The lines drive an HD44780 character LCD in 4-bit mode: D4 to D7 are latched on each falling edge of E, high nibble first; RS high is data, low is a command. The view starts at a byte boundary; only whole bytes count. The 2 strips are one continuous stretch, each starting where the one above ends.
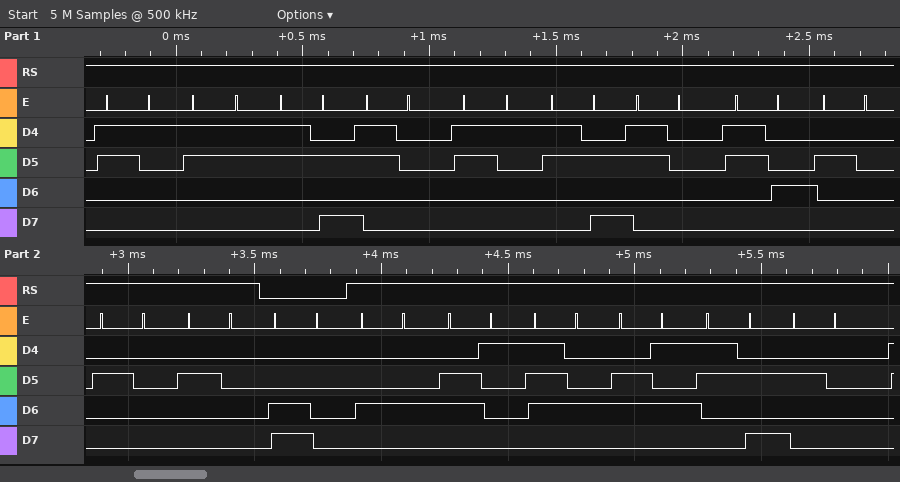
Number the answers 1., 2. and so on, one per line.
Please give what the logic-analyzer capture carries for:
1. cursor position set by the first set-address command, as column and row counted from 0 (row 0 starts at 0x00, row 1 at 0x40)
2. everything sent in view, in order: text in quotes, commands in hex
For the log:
1. column 0, row 1
2. "13:01:04   " 0xC0 "Date: "
